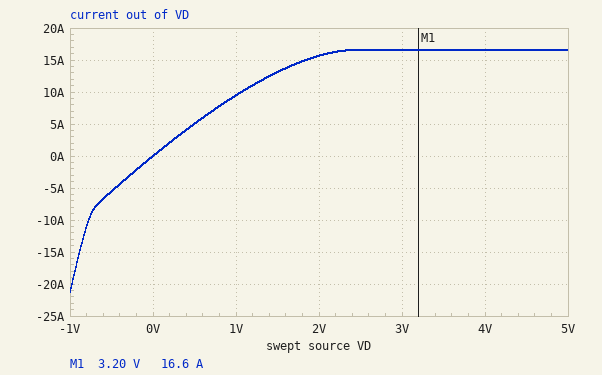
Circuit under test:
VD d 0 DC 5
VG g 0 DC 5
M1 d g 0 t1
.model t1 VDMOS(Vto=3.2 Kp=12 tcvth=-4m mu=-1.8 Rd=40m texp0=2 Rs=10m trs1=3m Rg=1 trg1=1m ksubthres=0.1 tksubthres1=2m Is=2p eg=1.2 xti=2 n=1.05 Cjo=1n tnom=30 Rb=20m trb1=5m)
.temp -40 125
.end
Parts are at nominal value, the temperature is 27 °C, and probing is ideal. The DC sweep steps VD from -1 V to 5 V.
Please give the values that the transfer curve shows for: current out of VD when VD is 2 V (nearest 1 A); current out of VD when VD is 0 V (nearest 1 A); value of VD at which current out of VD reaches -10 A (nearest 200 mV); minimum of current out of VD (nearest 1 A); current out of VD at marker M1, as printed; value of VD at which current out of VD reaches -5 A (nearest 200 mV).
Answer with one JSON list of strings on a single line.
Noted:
["16 A", "0 A", "-800 mV", "-21 A", "16.6 A", "-400 mV"]
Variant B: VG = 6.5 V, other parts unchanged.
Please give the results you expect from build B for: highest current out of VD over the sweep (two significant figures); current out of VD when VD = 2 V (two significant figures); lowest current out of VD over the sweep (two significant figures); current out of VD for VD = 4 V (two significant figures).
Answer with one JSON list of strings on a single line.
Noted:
["49 A", "25 A", "-24 A", "44 A"]
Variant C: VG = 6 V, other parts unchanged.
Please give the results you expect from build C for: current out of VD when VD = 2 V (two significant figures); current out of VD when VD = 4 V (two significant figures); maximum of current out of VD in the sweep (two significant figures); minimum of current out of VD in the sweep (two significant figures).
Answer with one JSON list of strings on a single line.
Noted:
["23 A", "36 A", "37 A", "-23 A"]
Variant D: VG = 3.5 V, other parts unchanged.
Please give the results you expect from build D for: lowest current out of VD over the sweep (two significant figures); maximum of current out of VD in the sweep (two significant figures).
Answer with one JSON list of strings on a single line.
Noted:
["-16 A", "590 mA"]
